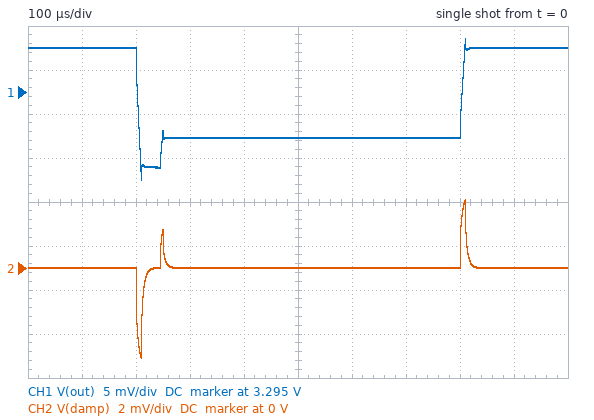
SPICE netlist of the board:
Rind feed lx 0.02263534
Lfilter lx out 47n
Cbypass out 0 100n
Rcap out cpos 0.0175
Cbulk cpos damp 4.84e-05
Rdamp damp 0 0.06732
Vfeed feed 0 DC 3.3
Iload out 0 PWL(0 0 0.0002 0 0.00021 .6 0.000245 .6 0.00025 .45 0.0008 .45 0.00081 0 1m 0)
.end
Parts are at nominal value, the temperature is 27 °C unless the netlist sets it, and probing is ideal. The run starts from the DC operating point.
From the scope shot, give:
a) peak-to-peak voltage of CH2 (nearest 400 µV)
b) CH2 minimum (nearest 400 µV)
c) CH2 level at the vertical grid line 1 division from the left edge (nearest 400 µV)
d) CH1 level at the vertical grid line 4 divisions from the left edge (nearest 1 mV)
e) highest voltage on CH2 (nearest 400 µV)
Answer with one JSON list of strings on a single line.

["7.2 mV", "-4.0 mV", "0 V", "3.290 V", "3.2 mV"]
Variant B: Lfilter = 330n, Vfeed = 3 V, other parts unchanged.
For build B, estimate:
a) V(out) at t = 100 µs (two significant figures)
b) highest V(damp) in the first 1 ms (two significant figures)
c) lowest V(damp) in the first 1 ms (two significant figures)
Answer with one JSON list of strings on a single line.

["3.0 V", "7.3 mV", "-9.7 mV"]
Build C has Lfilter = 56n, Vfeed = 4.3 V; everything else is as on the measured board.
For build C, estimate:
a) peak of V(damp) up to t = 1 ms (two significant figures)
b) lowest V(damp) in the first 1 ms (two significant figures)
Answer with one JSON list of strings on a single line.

["3.1 mV", "-4.2 mV"]
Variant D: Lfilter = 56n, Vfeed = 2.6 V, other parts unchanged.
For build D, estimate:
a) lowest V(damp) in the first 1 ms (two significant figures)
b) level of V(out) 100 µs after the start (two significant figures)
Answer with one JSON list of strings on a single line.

["-4.2 mV", "2.6 V"]
